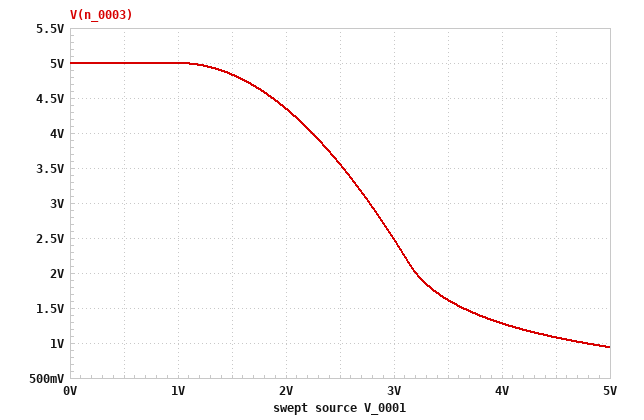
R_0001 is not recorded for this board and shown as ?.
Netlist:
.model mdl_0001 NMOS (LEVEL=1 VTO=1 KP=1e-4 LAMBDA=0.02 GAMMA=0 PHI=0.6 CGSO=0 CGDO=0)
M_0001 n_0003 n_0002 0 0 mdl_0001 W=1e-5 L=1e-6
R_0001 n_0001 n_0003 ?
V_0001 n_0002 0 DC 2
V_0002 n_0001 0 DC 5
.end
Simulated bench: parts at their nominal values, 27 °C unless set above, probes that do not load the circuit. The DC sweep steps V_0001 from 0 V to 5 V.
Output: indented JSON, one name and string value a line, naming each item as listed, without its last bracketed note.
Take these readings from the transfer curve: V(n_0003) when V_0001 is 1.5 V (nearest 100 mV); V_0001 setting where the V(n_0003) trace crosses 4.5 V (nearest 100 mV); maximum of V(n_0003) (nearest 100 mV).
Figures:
{
  "V(n_0003) when V_0001 is 1.5 V": "4.8 V",
  "V_0001 setting where the V(n_0003) trace crosses 4.5 V": "1.9 V",
  "maximum of V(n_0003)": "5.0 V"
}
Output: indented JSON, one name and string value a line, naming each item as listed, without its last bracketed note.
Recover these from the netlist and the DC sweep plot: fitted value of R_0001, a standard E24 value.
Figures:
{
  "fitted value of R_0001, a standard E24 value": "1.2 kΩ"
}
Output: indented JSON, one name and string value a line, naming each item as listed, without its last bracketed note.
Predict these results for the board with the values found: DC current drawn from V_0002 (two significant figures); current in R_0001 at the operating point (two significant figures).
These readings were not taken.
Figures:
{
  "DC current drawn from V_0002": "540 µA",
  "current in R_0001 at the operating point": "540 µA"
}
